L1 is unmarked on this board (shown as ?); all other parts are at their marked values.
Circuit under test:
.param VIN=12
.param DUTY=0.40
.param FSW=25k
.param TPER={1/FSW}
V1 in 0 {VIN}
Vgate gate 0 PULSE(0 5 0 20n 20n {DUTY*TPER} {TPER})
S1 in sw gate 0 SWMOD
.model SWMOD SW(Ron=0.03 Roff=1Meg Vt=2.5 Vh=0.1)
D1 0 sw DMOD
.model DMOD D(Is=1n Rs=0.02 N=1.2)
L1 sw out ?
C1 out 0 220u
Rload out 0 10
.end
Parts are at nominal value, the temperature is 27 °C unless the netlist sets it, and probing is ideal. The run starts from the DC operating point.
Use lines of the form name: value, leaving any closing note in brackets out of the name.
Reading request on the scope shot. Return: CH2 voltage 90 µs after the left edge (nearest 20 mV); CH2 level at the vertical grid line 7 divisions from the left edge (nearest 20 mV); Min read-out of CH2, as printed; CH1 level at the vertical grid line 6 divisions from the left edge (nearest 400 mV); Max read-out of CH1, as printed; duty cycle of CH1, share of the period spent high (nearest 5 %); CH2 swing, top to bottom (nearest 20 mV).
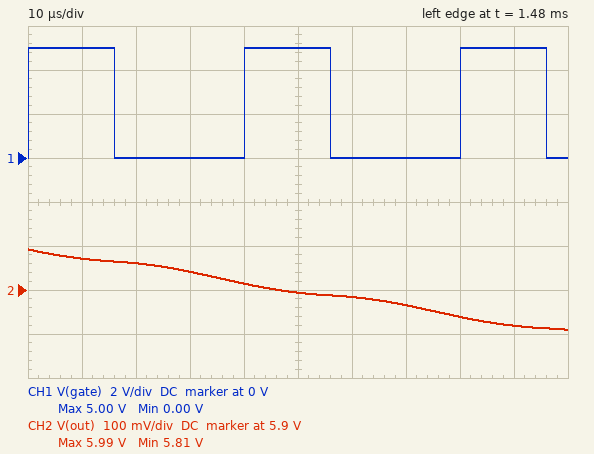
CH2 voltage 90 µs after the left edge: 5.82 V
CH2 level at the vertical grid line 7 divisions from the left edge: 5.86 V
Min read-out of CH2, as printed: 5.81 V
CH1 level at the vertical grid line 6 divisions from the left edge: 0 V
Max read-out of CH1, as printed: 5.00 V
duty cycle of CH1, share of the period spent high: 40 %
CH2 swing, top to bottom: 180 mV
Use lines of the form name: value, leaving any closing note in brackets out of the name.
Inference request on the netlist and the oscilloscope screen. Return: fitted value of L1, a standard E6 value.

fitted value of L1, a standard E6 value: 220 µH
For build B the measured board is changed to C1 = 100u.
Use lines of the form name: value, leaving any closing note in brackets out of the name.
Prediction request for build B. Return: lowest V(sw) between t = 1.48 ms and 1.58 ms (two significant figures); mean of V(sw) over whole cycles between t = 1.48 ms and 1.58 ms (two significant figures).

lowest V(sw) between t = 1.48 ms and 1.58 ms: -650 mV
mean of V(sw) over whole cycles between t = 1.48 ms and 1.58 ms: 4.4 V
